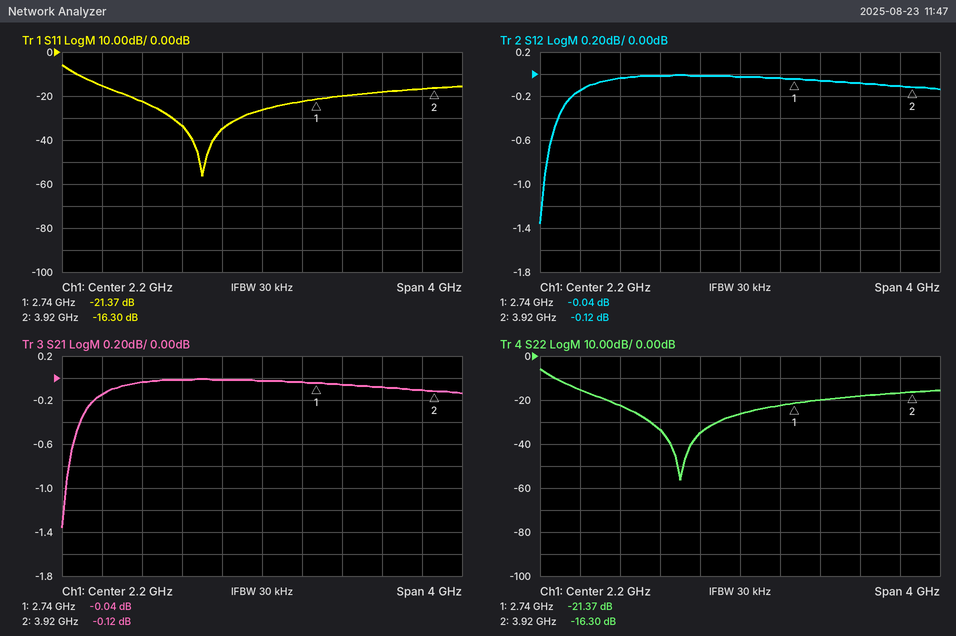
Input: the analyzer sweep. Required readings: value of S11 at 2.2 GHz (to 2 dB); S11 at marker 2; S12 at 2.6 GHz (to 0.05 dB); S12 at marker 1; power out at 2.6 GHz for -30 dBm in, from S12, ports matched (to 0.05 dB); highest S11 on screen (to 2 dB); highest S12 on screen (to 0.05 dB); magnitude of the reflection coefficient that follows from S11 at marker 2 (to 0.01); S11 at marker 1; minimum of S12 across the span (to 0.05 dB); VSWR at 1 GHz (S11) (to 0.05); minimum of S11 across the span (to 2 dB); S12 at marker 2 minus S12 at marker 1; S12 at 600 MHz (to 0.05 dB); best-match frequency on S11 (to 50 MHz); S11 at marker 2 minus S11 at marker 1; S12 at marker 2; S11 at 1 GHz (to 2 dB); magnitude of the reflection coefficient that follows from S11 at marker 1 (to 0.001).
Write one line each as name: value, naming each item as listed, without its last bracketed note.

value of S11 at 2.2 GHz: -26 dB
S11 at marker 2: -16.30 dB
S12 at 2.6 GHz: -0.05 dB
S12 at marker 1: -0.04 dB
power out at 2.6 GHz for -30 dBm in, from S12, ports matched: -30.05 dBm
highest S11 on screen: -6 dB
highest S12 on screen: 0.00 dB
magnitude of the reflection coefficient that follows from S11 at marker 2: 0.15
S11 at marker 1: -21.37 dB
minimum of S12 across the span: -1.35 dB
VSWR at 1 GHz (S11): 1.15
minimum of S11 across the span: -56 dB
S12 at marker 2 minus S12 at marker 1: -0.08 dB
S12 at 600 MHz: -0.15 dB
best-match frequency on S11: 1.60 GHz
S11 at marker 2 minus S11 at marker 1: 5.07 dB
S12 at marker 2: -0.12 dB
S11 at 1 GHz: -22 dB
magnitude of the reflection coefficient that follows from S11 at marker 1: 0.085
